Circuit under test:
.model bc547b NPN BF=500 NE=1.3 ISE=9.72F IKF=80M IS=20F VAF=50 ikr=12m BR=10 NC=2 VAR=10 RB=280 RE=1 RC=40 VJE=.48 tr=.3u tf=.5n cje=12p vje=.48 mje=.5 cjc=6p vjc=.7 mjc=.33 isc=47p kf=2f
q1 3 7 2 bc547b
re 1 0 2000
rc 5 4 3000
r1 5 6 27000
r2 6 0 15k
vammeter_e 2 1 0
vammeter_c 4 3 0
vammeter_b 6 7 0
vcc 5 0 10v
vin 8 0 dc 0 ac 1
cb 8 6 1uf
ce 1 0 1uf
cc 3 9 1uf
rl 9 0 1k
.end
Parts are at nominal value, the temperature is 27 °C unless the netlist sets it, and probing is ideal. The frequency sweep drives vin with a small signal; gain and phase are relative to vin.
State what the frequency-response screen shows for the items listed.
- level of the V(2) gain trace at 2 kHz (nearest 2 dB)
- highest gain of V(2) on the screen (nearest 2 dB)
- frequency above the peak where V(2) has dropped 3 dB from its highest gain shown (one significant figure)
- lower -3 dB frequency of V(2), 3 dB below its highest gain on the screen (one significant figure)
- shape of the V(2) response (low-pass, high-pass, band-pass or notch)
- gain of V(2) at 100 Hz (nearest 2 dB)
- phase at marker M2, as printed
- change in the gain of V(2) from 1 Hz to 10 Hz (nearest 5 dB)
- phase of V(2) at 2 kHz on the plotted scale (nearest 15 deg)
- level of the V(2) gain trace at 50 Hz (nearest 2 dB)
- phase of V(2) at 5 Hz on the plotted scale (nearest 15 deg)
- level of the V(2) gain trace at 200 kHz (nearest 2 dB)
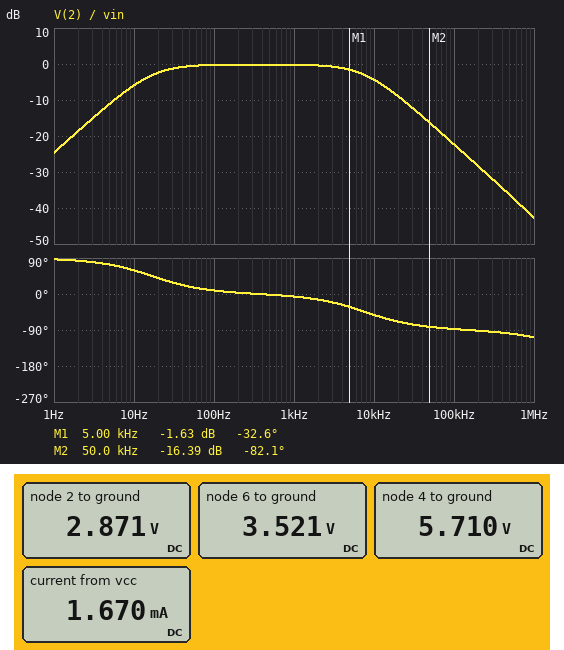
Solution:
0 dB
0 dB
8 kHz
20 Hz
band-pass
0 dB
-82.1 deg
20 dB
-15 deg
0 dB
75 deg
-28 dB
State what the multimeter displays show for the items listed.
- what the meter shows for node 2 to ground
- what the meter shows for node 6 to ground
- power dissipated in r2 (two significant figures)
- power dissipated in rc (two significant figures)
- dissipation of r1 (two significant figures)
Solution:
2.871 V
3.521 V
830 µW
6.1 mW
1.6 mW
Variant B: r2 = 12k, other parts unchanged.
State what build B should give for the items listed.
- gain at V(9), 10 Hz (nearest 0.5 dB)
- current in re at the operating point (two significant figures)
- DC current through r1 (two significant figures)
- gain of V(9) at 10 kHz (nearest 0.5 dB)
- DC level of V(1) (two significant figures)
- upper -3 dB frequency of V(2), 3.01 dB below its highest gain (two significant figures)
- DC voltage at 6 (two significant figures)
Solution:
-27.5 dB
1.2 mA
260 µA
28.0 dB
2.4 V
6.7 kHz
3.0 V
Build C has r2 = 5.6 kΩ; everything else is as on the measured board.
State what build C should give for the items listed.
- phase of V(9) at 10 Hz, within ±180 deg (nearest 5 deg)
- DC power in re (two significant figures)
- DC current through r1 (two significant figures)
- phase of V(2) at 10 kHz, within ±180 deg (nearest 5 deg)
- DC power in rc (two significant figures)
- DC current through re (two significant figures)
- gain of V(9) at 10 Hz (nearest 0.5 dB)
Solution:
-25 deg
590 µW
310 µA
-70 deg
880 µW
540 µA
-32.0 dB
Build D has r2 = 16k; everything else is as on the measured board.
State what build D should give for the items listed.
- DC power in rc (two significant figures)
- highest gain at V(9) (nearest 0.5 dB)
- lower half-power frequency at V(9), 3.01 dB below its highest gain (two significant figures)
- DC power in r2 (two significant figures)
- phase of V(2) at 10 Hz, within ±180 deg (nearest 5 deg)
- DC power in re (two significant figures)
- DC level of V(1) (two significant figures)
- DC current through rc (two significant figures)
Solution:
6.8 mW
31.5 dB
8.1 kHz
840 µW
60 deg
4.5 mW
3.0 V
1.5 mA
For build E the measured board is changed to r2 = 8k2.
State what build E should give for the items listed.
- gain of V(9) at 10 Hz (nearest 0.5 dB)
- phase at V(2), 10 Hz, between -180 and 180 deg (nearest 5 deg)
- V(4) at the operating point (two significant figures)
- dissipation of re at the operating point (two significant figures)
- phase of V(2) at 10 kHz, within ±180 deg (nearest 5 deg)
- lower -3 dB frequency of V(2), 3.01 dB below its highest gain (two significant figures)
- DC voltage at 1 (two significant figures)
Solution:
-29.5 dB
70 deg
7.5 V
1.4 mW
-65 deg
25 Hz
1.7 V
